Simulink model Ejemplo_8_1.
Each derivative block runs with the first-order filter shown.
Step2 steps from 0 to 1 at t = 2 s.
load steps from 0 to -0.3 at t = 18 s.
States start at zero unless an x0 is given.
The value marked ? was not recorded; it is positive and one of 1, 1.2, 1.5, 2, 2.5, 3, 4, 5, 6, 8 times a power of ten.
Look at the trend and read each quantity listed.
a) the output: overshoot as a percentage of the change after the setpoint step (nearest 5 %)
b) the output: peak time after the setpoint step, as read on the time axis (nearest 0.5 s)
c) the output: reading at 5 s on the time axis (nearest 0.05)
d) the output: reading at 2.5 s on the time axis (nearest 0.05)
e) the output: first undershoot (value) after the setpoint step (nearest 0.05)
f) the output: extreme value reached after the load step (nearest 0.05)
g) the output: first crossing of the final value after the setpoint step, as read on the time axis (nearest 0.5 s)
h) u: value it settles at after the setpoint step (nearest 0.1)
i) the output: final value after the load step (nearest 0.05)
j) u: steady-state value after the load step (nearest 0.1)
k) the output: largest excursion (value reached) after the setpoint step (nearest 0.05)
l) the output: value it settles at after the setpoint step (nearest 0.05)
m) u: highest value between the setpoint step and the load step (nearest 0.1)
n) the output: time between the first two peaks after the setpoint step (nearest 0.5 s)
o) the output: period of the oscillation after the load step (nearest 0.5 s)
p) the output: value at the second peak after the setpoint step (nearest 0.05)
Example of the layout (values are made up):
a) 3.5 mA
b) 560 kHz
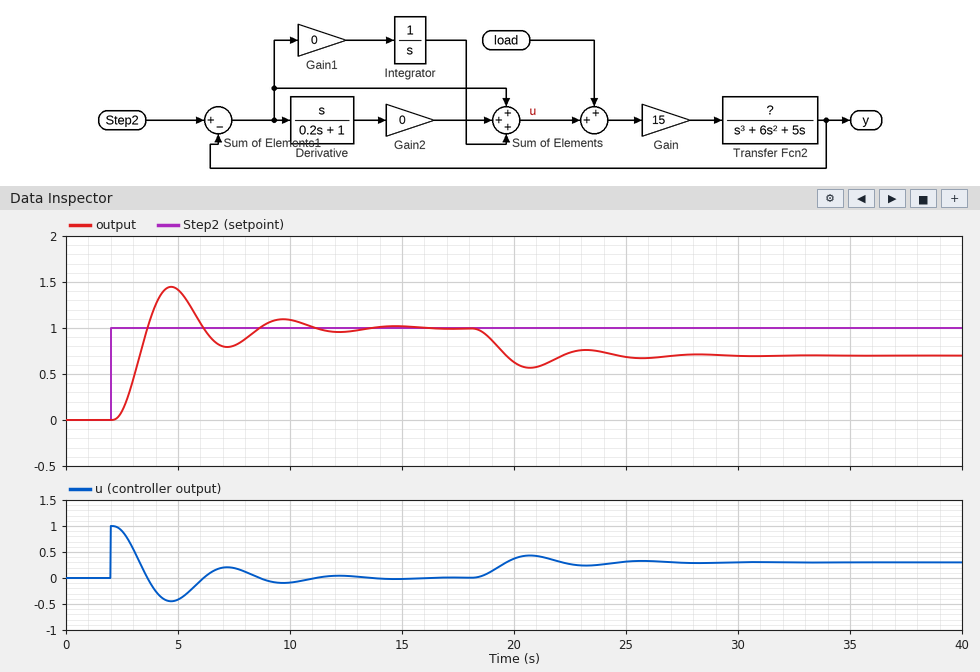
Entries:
a) 45 %
b) 4.5 s
c) 1.40
d) 0.10
e) 0.80
f) 0.55
g) 3.5 s
h) 0.0
i) 0.70
j) 0.3
k) 1.45
l) 1.00
m) 1.0
n) 5.0 s
o) 5.0 s
p) 1.10
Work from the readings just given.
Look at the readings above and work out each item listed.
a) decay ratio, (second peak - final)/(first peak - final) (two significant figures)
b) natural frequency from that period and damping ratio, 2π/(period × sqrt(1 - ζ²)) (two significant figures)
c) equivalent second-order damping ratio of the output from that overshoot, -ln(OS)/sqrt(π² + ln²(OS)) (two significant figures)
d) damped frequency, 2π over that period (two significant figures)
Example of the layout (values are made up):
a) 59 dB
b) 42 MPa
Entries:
a) 0.22
b) 1.3 rad/s
c) 0.25
d) 1.3 rad/s
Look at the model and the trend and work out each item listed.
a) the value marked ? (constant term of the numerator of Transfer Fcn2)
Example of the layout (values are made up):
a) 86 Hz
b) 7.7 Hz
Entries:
a) 0.6
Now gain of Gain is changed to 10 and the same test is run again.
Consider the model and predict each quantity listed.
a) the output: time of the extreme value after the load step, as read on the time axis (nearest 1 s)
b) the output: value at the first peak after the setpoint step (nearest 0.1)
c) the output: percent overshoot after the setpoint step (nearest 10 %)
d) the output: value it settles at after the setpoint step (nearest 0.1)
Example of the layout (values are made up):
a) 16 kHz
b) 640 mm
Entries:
a) 21 s
b) 1.3
c) 30 %
d) 1.0
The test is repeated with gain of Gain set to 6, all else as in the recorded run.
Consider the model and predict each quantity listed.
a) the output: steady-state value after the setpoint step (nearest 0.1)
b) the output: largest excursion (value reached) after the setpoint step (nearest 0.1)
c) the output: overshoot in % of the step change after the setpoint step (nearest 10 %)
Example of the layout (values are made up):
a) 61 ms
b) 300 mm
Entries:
a) 1.0
b) 1.2
c) 20 %
